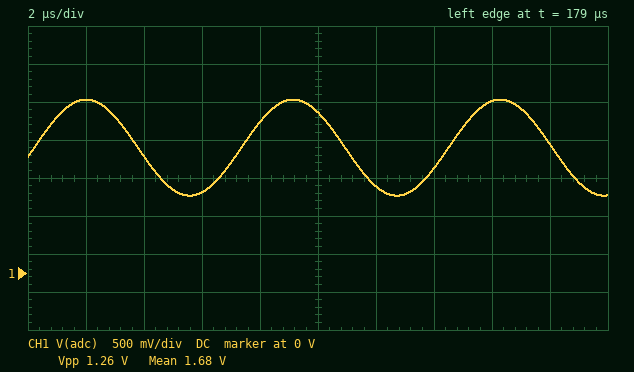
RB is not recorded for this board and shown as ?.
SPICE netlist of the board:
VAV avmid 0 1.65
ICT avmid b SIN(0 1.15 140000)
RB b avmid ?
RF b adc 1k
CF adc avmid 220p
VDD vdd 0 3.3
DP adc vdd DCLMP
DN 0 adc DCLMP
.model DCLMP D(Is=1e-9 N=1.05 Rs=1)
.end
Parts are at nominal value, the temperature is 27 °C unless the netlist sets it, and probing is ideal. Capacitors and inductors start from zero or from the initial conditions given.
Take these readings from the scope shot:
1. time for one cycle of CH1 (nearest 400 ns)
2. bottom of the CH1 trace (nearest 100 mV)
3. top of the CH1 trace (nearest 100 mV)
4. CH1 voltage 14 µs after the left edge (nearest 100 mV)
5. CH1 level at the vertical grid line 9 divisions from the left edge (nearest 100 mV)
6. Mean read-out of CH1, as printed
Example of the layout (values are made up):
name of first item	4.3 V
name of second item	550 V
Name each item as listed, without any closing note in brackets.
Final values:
time for one cycle of CH1	7.2 µs
bottom of the CH1 trace	1.0 V
top of the CH1 trace	2.3 V
CH1 voltage 14 µs after the left edge	1.4 V
CH1 level at the vertical grid line 9 divisions from the left edge	1.7 V
Mean read-out of CH1, as printed	1.68 V
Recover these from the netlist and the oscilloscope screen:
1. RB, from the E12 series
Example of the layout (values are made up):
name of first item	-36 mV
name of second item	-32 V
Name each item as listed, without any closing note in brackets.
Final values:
RB, from the E12 series	0.56 Ω
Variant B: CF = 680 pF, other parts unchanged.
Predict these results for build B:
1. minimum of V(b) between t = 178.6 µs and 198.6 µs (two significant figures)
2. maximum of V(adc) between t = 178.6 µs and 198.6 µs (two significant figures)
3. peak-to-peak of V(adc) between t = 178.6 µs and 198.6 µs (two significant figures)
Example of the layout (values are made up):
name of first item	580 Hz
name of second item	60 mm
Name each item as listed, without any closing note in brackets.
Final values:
minimum of V(b) between t = 178.6 µs and 198.6 µs	1.0 V
maximum of V(adc) between t = 178.6 µs and 198.6 µs	2.2 V
peak-to-peak of V(adc) between t = 178.6 µs and 198.6 µs	1.1 V
